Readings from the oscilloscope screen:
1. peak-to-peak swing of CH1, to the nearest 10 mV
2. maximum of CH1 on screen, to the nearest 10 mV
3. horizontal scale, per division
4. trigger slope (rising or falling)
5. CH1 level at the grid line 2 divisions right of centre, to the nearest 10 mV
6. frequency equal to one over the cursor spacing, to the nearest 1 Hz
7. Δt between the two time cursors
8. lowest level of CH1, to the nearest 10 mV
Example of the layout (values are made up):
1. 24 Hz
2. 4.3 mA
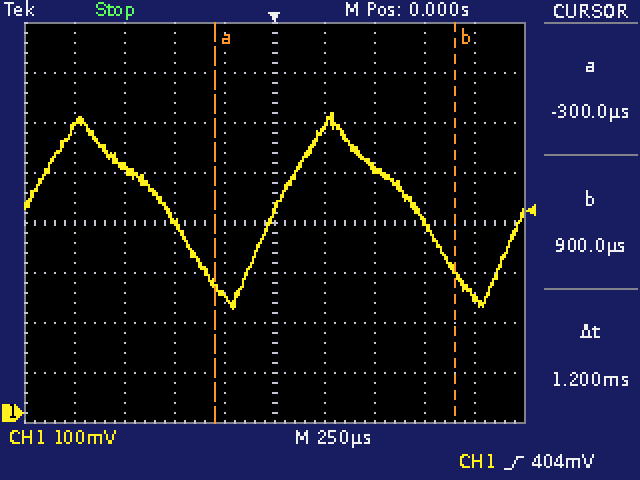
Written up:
1. 390 mV
2. 600 mV
3. 250 µs
4. rising
5. 490 mV
6. 833 Hz
7. 1.2 ms
8. 210 mV
